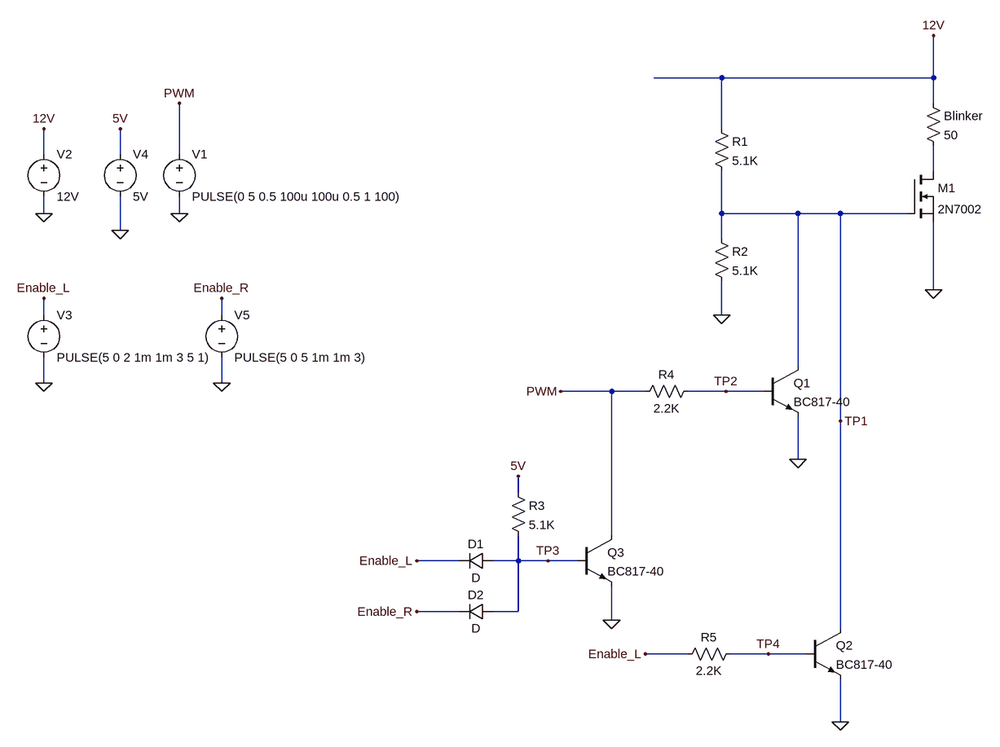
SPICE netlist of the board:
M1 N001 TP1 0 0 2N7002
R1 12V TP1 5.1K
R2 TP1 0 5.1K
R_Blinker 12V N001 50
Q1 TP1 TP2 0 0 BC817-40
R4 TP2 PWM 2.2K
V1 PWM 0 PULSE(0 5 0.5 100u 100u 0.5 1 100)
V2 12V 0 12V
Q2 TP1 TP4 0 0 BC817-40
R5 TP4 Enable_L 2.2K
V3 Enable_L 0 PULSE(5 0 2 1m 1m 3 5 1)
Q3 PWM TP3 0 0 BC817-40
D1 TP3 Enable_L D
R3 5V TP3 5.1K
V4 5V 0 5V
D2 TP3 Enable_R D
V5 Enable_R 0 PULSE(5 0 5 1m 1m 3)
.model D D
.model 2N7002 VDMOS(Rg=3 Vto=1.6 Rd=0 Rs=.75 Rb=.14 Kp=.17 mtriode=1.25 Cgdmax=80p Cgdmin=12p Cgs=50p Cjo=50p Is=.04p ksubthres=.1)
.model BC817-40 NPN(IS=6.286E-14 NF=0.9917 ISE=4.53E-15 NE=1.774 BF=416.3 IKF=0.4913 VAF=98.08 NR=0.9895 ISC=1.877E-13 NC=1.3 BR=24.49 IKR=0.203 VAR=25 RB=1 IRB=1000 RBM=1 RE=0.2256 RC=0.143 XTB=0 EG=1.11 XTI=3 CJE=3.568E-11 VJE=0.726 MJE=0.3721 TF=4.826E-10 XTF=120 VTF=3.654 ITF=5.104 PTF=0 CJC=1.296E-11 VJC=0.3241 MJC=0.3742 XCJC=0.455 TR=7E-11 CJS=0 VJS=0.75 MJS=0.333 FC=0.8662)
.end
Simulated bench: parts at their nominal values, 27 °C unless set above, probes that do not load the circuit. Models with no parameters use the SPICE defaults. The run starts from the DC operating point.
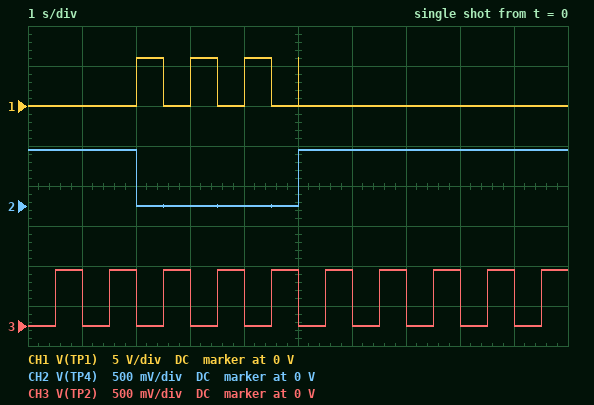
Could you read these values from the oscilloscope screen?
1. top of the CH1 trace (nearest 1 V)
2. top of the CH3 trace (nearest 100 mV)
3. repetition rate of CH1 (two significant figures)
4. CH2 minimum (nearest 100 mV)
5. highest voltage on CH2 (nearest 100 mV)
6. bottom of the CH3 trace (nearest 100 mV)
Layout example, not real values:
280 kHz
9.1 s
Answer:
6 V
700 mV
1.0 Hz
0 V
700 mV
0 V
